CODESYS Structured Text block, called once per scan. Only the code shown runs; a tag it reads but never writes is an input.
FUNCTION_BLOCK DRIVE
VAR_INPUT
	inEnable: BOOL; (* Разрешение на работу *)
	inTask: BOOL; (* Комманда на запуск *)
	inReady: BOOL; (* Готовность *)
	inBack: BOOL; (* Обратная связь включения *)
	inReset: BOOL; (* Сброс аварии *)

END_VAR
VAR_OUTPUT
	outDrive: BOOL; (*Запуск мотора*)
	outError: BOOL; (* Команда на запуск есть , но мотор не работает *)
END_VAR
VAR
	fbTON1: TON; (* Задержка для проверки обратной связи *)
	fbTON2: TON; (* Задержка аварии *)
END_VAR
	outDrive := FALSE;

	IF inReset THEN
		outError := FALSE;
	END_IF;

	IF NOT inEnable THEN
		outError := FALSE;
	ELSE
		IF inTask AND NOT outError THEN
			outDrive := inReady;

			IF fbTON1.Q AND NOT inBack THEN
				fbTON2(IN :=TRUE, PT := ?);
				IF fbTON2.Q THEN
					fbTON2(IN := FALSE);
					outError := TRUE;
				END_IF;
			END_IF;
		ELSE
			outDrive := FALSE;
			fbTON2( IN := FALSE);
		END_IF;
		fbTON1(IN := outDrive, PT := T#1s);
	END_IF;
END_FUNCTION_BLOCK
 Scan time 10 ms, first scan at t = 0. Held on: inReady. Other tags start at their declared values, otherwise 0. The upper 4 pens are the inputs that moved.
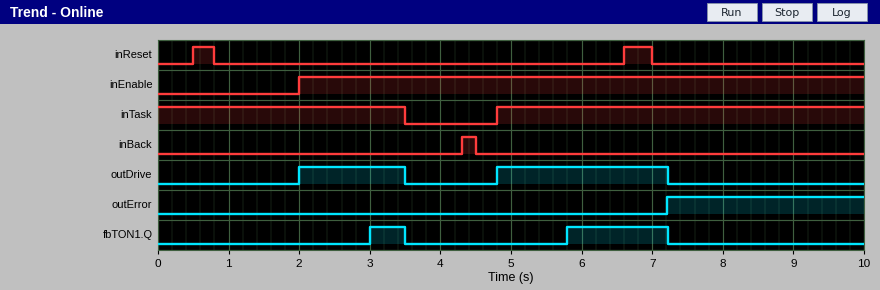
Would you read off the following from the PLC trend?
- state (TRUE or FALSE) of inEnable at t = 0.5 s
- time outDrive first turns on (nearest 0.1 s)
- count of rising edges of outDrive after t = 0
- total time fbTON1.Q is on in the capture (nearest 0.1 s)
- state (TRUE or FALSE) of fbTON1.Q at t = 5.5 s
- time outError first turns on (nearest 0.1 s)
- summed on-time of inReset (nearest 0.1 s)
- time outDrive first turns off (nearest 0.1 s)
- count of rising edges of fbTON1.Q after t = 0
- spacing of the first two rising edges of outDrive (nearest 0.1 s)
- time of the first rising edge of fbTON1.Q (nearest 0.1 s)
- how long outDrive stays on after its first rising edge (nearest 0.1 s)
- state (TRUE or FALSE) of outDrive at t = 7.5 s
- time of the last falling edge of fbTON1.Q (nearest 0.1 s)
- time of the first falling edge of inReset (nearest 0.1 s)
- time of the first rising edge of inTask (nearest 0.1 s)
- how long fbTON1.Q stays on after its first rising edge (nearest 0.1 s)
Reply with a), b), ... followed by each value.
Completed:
a) FALSE
b) 2.0 s
c) 2
d) 1.9 s
e) FALSE
f) 7.2 s
g) 0.7 s
h) 3.5 s
i) 2
j) 2.8 s
k) 3.0 s
l) 1.5 s
m) FALSE
n) 7.2 s
o) 0.8 s
p) 4.8 s
q) 0.5 s
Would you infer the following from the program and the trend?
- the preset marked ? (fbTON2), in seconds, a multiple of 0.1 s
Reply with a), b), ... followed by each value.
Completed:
a) 1.4 s
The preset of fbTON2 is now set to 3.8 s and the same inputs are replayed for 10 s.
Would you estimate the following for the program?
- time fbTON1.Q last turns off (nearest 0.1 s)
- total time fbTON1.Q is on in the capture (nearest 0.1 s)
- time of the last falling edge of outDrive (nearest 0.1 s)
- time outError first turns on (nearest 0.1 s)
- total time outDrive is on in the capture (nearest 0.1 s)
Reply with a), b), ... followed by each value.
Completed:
a) 9.6 s
b) 4.3 s
c) 9.6 s
d) 9.6 s
e) 6.3 s
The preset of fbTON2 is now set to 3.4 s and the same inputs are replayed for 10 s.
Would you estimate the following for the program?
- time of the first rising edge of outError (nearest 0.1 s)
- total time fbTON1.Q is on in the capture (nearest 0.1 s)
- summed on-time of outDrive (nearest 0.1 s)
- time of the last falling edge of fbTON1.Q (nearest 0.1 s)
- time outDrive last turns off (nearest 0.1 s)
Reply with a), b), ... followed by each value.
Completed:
a) 9.2 s
b) 3.9 s
c) 5.9 s
d) 9.2 s
e) 9.2 s
